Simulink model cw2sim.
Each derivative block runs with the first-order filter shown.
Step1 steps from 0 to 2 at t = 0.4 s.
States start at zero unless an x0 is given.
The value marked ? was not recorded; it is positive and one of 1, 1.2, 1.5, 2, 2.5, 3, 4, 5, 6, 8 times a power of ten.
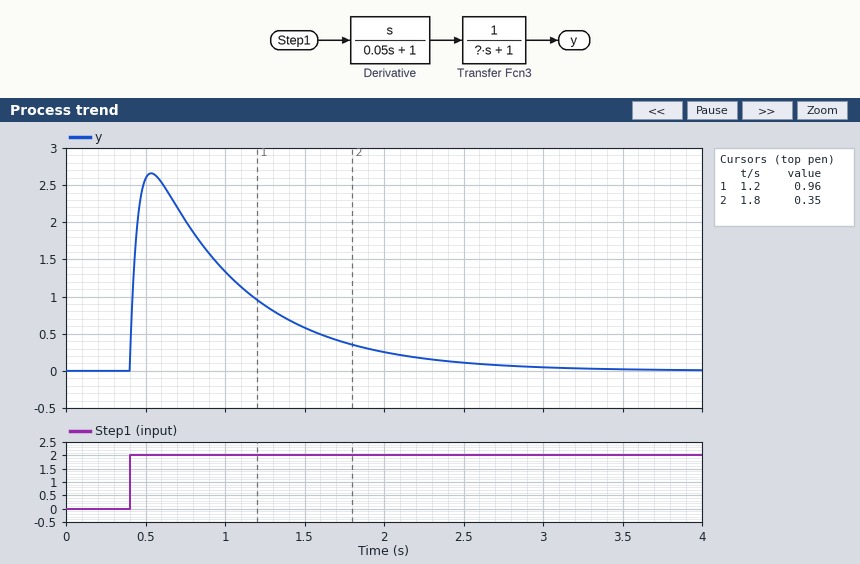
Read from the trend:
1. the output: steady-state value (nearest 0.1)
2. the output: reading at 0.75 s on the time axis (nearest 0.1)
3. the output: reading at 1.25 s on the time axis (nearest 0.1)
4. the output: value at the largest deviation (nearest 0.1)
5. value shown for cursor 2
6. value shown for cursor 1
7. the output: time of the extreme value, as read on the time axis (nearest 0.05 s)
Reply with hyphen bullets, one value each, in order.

- 0.0
- 2.0
- 0.9
- 2.7
- 0.35
- 0.96
- 0.55 s
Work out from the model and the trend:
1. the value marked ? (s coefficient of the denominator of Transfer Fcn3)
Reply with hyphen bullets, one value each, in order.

- 0.6
